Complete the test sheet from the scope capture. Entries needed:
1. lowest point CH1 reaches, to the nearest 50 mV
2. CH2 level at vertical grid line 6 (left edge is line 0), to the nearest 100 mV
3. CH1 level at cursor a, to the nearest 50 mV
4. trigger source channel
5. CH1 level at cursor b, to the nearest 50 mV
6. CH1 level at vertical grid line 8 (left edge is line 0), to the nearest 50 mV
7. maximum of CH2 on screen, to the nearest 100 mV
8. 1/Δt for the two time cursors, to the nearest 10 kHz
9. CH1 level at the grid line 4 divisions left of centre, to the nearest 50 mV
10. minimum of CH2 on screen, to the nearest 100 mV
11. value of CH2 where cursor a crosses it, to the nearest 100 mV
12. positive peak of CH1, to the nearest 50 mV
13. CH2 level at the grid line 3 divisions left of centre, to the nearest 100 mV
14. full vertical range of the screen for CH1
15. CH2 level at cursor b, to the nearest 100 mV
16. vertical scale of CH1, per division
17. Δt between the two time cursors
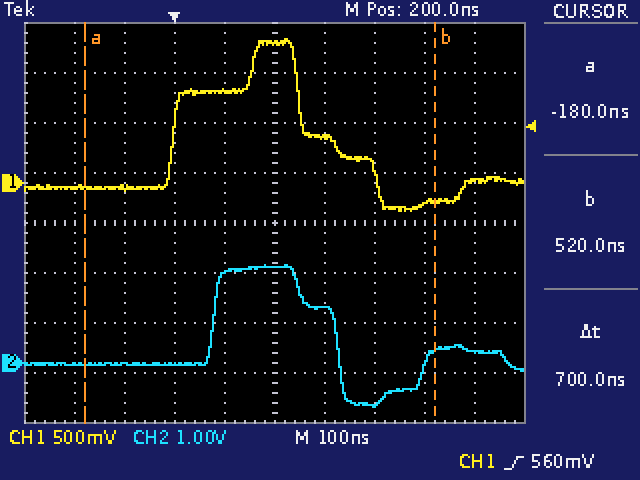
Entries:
-300 mV
1.1 V
-50 mV
CH1
-200 mV
-200 mV
2.0 V
1.43 MHz
-50 mV
-900 mV
0.0 V
1.45 V
0.0 V
4 V
200 mV
500 mV
700 ns
